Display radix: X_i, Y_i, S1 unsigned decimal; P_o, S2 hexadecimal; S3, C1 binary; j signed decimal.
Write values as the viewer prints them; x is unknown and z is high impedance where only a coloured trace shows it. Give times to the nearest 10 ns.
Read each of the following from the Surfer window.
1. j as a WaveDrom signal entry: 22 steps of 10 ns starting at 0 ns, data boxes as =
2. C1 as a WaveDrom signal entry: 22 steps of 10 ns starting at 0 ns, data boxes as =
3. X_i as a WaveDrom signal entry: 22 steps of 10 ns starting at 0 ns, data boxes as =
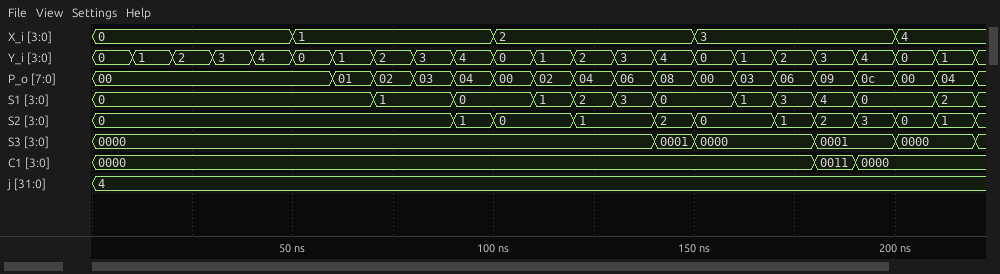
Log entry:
{name: 'j', wave: '=.....................', data: '4'}
{name: 'C1', wave: '=.................==..', data: '0000 0011 0000'}
{name: 'X_i', wave: '=....=....=....=....=.', data: '0 1 2 3 4'}
